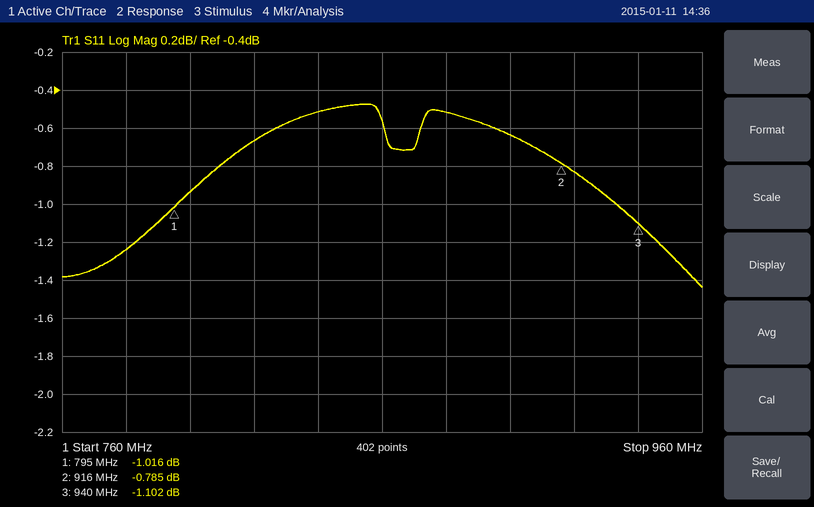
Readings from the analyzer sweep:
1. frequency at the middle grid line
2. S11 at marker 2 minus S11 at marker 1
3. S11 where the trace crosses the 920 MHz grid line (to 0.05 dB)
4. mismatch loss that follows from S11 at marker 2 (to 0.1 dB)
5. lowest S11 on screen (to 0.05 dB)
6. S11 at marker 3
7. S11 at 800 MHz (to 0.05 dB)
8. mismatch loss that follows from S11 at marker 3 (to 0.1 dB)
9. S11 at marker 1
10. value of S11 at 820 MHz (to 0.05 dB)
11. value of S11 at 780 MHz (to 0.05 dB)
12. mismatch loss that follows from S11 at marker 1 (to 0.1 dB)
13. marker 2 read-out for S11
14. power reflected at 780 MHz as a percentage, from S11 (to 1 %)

860 MHz
0.231 dB
-0.85 dB
7.8 dB
-1.45 dB
-1.102 dB
-0.95 dB
6.5 dB
-1.016 dB
-0.65 dB
-1.25 dB
6.8 dB
-0.785 dB
75 %
